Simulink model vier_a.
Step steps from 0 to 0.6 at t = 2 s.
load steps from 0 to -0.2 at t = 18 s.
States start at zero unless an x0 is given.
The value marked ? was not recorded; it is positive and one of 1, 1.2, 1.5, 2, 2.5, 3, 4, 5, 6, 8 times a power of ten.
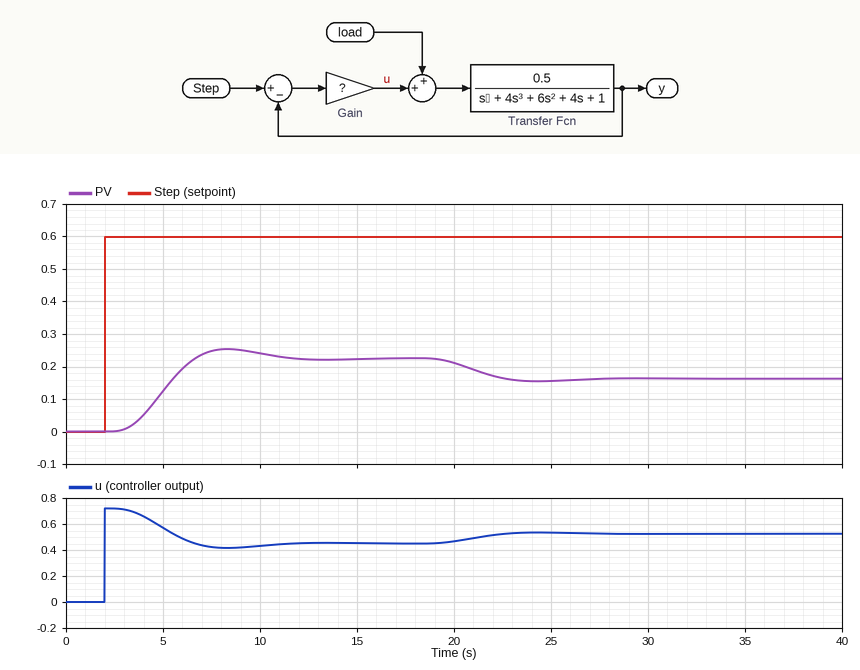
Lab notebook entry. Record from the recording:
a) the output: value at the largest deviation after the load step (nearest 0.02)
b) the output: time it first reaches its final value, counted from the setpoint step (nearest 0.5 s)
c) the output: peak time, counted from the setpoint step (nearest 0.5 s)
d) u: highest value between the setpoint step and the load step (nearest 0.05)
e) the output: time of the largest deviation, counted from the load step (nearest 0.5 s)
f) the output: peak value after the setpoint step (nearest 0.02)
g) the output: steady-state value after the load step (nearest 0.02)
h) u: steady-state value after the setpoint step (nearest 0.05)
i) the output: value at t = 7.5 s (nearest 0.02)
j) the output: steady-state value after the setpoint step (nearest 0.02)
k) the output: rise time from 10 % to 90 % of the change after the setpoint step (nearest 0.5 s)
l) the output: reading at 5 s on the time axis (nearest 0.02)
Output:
0.16
4.5 s
6.5 s
0.70
6.5 s
0.26
0.16
0.45
0.24
0.22
2.5 s
0.12
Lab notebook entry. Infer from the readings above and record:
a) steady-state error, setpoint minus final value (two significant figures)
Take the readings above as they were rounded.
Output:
0.38
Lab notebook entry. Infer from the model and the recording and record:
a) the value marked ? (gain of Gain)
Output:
1.2
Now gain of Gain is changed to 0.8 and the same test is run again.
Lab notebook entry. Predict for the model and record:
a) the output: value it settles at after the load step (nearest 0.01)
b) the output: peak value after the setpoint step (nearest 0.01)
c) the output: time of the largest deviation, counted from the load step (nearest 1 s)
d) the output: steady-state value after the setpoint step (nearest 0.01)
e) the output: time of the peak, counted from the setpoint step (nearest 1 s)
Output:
0.10
0.18
7 s
0.17
7 s
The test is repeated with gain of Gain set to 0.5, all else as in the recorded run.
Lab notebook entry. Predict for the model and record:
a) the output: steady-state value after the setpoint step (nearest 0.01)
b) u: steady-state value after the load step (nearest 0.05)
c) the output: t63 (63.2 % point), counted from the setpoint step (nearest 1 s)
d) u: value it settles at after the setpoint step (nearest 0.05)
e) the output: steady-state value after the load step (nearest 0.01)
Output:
0.12
0.30
4 s
0.25
0.04
